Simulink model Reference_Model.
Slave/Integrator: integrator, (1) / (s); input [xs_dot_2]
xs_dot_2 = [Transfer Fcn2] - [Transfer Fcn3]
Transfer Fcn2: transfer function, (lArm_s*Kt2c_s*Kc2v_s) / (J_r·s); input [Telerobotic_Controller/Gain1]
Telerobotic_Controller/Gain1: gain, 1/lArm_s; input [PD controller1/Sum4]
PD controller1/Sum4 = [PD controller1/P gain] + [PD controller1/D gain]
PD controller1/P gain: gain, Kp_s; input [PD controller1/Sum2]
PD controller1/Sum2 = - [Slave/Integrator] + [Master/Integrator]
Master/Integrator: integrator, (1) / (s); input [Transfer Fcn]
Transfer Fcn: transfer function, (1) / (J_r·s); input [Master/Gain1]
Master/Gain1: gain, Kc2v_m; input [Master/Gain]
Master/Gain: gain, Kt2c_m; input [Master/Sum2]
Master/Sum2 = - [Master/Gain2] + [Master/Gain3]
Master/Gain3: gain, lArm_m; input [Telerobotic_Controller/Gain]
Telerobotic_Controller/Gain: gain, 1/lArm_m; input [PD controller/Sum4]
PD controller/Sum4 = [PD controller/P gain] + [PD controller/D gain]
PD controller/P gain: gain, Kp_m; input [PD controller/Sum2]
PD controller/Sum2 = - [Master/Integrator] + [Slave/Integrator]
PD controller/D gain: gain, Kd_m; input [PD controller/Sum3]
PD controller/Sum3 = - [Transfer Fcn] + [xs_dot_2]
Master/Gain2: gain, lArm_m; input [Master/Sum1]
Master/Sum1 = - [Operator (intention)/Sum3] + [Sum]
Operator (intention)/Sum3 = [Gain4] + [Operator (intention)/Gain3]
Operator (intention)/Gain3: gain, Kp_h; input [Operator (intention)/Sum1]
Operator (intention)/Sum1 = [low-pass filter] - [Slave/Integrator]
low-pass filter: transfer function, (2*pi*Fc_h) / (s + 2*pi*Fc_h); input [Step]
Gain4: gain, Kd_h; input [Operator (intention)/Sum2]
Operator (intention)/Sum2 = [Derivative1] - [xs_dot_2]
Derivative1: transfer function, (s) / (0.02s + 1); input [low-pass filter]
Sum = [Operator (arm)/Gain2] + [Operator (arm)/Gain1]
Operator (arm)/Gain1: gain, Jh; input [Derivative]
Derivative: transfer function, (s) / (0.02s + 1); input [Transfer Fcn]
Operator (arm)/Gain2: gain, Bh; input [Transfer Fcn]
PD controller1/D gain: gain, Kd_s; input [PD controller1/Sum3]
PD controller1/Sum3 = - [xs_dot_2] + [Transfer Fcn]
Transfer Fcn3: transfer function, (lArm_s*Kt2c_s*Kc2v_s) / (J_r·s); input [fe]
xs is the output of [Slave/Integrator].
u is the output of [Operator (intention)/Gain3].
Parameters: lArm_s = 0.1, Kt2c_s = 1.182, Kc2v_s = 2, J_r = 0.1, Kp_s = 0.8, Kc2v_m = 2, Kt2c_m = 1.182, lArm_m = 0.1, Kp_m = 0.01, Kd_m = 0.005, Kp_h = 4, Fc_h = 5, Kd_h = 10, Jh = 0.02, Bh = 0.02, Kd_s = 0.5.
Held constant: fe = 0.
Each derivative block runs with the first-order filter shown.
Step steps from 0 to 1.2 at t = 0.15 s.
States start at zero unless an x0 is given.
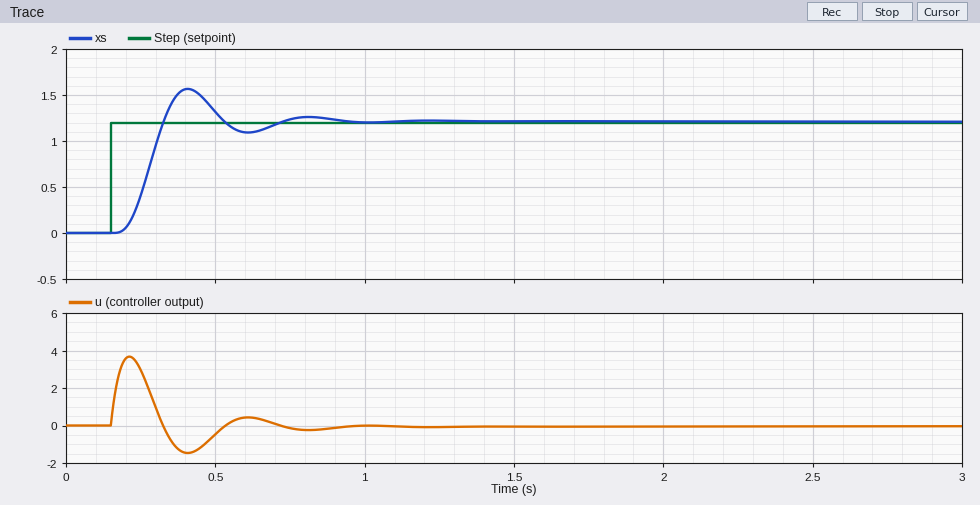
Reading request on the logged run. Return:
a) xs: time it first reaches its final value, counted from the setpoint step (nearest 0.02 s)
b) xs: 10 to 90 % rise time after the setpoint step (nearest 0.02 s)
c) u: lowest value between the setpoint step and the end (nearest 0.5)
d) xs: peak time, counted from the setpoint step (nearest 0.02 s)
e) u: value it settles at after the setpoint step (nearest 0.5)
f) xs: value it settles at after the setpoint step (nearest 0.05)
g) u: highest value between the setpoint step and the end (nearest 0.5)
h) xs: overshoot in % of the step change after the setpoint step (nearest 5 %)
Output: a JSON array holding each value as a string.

["0.18 s", "0.10 s", "-1.5", "0.26 s", "0.0", "1.20", "3.5", "30 %"]
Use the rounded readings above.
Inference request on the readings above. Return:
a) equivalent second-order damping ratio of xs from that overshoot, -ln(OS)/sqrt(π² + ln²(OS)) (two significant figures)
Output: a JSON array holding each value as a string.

["0.36"]
